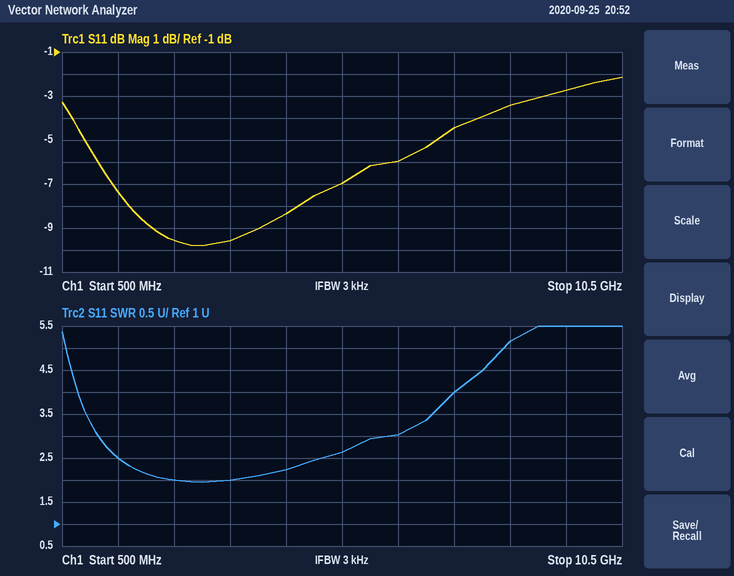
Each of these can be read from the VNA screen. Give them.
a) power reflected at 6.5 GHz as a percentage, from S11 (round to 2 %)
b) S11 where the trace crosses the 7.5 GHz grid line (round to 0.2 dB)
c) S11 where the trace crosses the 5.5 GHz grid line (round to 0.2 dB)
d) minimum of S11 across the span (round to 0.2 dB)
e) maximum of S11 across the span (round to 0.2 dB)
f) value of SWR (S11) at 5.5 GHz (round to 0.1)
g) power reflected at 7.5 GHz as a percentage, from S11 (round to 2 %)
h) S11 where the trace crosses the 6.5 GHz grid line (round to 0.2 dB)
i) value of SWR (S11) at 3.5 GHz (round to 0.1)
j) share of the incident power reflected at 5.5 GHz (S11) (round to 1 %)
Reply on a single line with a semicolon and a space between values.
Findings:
26 %; -4.4 dB; -7.0 dB; -9.8 dB; -2.2 dB; 2.6; 36 %; -6.0 dB; 2.0; 20 %
